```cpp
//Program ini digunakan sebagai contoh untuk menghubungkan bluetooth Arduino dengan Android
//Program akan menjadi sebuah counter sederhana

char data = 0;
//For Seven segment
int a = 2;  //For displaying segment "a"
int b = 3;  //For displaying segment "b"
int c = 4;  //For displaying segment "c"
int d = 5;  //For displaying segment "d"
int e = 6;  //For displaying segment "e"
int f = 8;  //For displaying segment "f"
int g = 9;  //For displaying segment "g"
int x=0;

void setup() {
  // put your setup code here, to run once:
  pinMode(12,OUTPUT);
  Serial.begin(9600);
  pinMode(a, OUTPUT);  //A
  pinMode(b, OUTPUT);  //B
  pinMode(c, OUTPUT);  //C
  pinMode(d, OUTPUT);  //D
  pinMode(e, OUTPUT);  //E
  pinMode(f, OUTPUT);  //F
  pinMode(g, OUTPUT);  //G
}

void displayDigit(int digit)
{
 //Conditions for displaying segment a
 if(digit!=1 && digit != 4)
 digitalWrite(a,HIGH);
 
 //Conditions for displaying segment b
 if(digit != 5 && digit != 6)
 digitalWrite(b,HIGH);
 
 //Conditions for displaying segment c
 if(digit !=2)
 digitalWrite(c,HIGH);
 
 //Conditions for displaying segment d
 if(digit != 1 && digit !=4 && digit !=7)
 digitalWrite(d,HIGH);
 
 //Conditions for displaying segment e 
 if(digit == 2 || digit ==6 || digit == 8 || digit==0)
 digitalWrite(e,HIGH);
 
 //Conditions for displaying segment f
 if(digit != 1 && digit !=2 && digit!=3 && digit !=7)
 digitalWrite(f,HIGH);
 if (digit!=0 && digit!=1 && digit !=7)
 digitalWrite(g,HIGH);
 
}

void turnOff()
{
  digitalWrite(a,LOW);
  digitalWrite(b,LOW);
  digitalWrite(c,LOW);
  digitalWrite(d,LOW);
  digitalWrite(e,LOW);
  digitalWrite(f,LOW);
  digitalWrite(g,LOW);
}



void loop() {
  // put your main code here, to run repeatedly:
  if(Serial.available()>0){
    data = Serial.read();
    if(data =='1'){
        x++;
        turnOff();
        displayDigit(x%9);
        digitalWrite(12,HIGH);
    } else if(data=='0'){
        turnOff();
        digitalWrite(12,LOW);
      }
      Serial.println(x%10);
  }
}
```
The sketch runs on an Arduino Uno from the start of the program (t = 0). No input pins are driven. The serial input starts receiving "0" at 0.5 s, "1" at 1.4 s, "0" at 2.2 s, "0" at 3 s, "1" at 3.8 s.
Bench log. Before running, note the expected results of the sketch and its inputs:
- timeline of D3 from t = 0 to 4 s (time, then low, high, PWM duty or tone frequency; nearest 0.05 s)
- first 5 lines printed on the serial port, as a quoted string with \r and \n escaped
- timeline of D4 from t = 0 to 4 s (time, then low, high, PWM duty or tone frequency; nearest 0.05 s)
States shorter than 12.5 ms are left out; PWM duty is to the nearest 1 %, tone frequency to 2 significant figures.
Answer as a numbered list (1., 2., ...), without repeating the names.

1. 0 s low; 1.4 s high; 2.2 s low; 3.8 s high
2. "0\r\n1\r\n1\r\n1\r\n2\r\n"
3. 0 s low; 1.4 s high; 2.2 s low
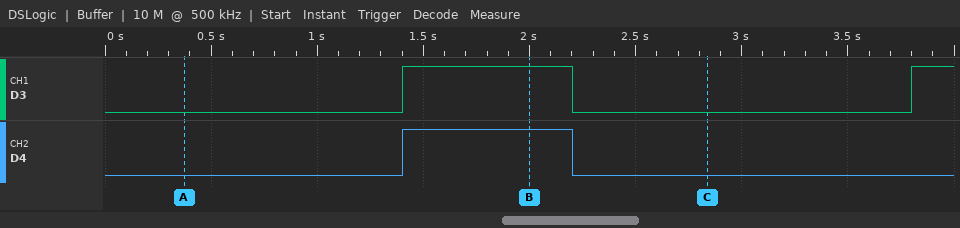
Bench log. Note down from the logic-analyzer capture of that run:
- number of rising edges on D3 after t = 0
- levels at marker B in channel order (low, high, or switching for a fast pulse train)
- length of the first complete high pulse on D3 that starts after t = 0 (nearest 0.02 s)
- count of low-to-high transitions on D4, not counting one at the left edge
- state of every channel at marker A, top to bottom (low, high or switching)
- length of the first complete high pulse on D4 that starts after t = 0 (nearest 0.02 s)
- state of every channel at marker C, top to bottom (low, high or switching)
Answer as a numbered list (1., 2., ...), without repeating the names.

1. 2
2. D3 high, D4 high
3. 0.80 s
4. 1
5. D3 low, D4 low
6. 0.80 s
7. D3 low, D4 low
